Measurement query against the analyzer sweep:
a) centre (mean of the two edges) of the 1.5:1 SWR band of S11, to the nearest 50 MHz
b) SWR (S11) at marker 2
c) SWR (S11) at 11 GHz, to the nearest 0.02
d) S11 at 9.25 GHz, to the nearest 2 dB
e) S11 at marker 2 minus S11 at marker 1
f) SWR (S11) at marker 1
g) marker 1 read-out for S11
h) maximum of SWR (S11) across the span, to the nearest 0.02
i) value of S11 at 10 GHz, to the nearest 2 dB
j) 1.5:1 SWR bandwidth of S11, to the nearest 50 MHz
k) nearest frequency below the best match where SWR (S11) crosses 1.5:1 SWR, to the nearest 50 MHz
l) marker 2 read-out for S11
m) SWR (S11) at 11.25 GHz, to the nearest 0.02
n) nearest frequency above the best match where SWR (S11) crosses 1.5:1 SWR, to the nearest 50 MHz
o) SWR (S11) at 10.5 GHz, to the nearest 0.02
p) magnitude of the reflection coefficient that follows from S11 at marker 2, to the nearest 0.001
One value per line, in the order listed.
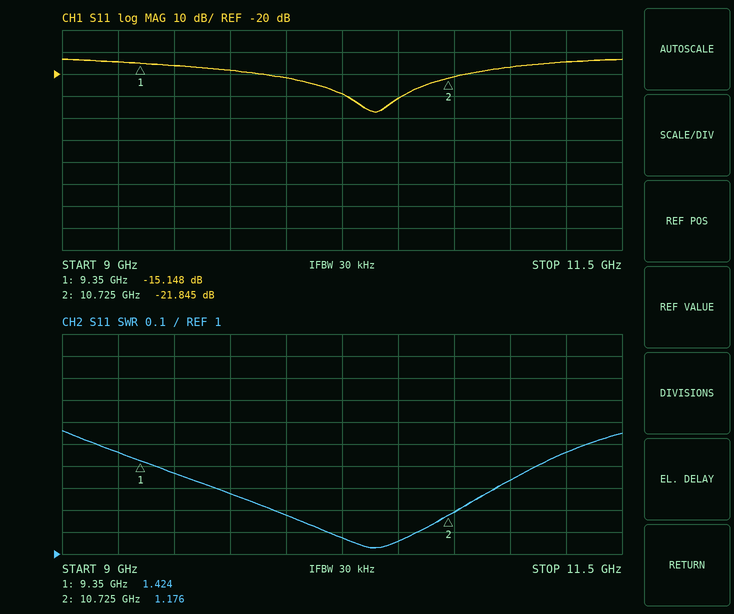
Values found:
10.25 GHz
1.176
1.34
-14 dB
-6.697 dB
1.424
-15.148 dB
1.56
-22 dB
2.20 GHz
9.15 GHz
-21.845 dB
1.46
11.35 GHz
1.06
0.081
